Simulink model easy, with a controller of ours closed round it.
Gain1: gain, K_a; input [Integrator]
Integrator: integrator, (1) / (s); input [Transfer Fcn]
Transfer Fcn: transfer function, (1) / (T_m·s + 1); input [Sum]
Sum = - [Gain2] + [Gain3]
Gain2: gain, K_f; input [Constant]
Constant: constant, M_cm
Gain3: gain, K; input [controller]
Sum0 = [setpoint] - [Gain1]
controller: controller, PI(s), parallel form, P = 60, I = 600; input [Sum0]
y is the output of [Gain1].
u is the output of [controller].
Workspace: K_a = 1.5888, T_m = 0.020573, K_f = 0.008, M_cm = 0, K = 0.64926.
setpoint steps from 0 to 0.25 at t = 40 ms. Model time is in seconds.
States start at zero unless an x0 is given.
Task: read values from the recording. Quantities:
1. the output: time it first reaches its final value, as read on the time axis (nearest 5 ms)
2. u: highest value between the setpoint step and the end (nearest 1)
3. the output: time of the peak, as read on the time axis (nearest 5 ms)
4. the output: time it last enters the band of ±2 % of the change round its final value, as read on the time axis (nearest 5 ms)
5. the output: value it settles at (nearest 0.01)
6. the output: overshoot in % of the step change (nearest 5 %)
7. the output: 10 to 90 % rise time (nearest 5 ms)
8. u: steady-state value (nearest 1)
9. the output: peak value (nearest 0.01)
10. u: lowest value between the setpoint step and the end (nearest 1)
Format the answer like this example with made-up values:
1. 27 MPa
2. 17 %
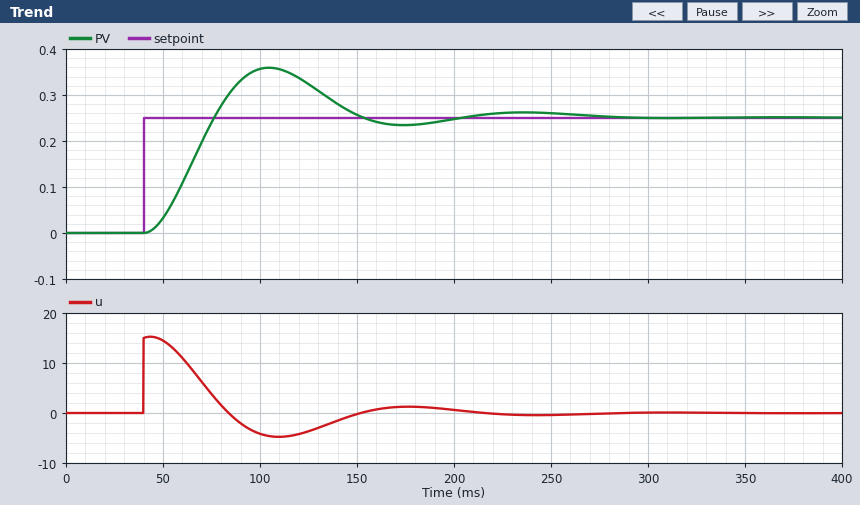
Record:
1. 75 ms
2. 15
3. 105 ms
4. 270 ms
5. 0.25
6. 45 %
7. 25 ms
8. 0
9. 0.36
10. -5
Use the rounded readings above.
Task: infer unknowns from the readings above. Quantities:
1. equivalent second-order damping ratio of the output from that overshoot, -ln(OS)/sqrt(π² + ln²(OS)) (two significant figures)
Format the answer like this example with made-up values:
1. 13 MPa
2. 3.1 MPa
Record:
1. 0.25
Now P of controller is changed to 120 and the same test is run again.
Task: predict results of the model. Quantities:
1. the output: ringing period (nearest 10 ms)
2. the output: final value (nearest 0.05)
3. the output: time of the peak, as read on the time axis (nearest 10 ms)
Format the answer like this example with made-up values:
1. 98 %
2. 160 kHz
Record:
1. 90 ms
2. 0.25
3. 80 ms
